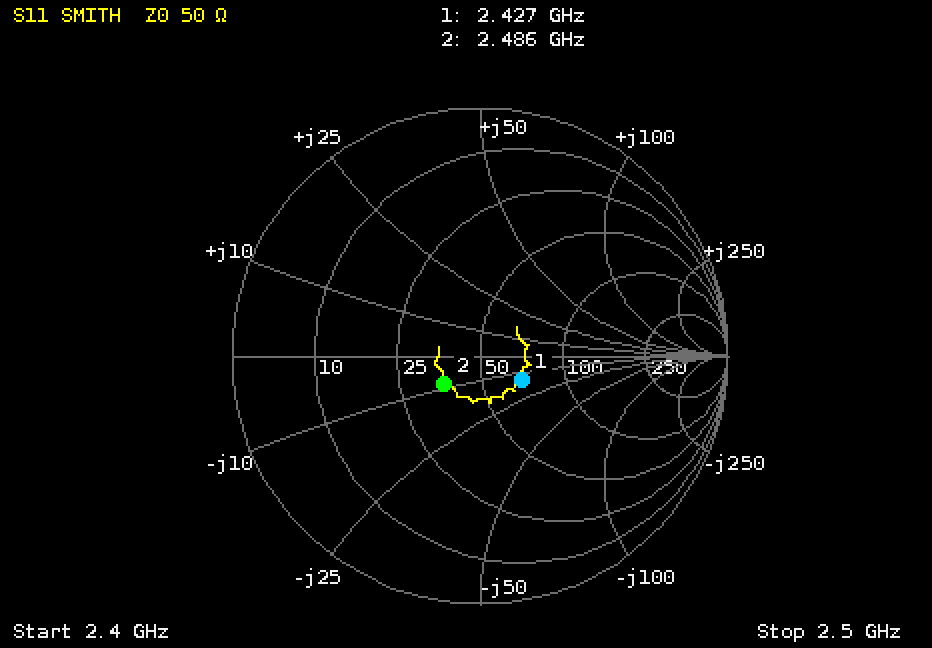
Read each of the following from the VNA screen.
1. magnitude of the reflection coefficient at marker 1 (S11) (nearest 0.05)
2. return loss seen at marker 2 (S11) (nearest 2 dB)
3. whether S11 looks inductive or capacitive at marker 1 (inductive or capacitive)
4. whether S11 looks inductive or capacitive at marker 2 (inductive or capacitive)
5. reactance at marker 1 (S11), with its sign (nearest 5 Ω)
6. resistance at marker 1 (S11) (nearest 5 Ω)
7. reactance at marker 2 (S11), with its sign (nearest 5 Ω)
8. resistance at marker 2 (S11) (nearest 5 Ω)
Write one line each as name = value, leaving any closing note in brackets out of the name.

magnitude of the reflection coefficient at marker 1 (S11) = 0.20
return loss seen at marker 2 (S11) = 14 dB
whether S11 looks inductive or capacitive at marker 1 = capacitive
whether S11 looks inductive or capacitive at marker 2 = capacitive
reactance at marker 1 (S11), with its sign = -15 Ω
resistance at marker 1 (S11) = 70 Ω
reactance at marker 2 (S11), with its sign = -10 Ω
resistance at marker 2 (S11) = 35 Ω
